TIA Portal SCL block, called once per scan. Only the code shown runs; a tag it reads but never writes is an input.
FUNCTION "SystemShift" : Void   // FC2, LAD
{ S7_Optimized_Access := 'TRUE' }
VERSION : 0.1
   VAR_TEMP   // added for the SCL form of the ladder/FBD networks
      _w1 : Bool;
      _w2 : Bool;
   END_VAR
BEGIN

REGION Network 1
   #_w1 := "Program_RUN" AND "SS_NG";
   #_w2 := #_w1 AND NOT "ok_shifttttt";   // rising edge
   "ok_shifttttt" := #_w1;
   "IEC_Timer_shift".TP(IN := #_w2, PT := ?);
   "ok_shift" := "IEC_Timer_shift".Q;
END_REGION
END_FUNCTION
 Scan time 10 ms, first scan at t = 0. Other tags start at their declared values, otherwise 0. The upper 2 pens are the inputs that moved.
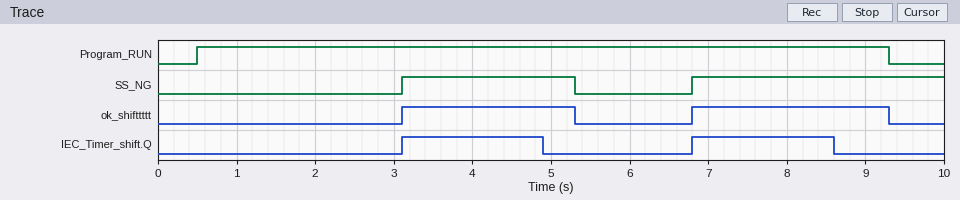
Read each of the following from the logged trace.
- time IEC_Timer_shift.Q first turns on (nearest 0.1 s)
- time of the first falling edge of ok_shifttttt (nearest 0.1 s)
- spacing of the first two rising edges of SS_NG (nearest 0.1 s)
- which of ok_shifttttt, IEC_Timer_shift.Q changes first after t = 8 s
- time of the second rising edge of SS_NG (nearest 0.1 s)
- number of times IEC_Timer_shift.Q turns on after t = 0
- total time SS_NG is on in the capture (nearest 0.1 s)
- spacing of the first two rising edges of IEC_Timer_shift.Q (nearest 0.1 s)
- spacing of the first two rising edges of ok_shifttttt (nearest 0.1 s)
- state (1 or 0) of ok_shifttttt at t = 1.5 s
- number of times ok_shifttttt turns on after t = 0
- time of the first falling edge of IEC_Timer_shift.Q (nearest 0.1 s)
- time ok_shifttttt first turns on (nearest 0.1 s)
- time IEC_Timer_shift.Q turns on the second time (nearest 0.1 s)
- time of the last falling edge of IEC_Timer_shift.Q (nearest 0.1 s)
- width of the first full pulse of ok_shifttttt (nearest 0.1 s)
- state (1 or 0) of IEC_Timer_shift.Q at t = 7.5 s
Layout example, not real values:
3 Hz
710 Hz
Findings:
3.1 s
5.3 s
3.7 s
IEC_Timer_shift.Q
6.8 s
2
5.4 s
3.7 s
3.7 s
0
2
4.9 s
3.1 s
6.8 s
8.6 s
2.2 s
1
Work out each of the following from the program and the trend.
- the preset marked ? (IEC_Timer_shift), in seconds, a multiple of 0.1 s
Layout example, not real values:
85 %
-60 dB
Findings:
1.8 s
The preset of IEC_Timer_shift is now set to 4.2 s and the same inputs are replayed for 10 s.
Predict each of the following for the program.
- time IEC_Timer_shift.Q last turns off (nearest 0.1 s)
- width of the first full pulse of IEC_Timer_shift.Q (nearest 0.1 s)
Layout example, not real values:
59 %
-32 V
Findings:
7.3 s
4.2 s
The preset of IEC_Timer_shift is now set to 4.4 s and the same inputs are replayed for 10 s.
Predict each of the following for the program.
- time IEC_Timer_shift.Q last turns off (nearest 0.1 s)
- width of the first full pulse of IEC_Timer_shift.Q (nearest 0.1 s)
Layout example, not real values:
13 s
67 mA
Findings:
7.5 s
4.4 s
